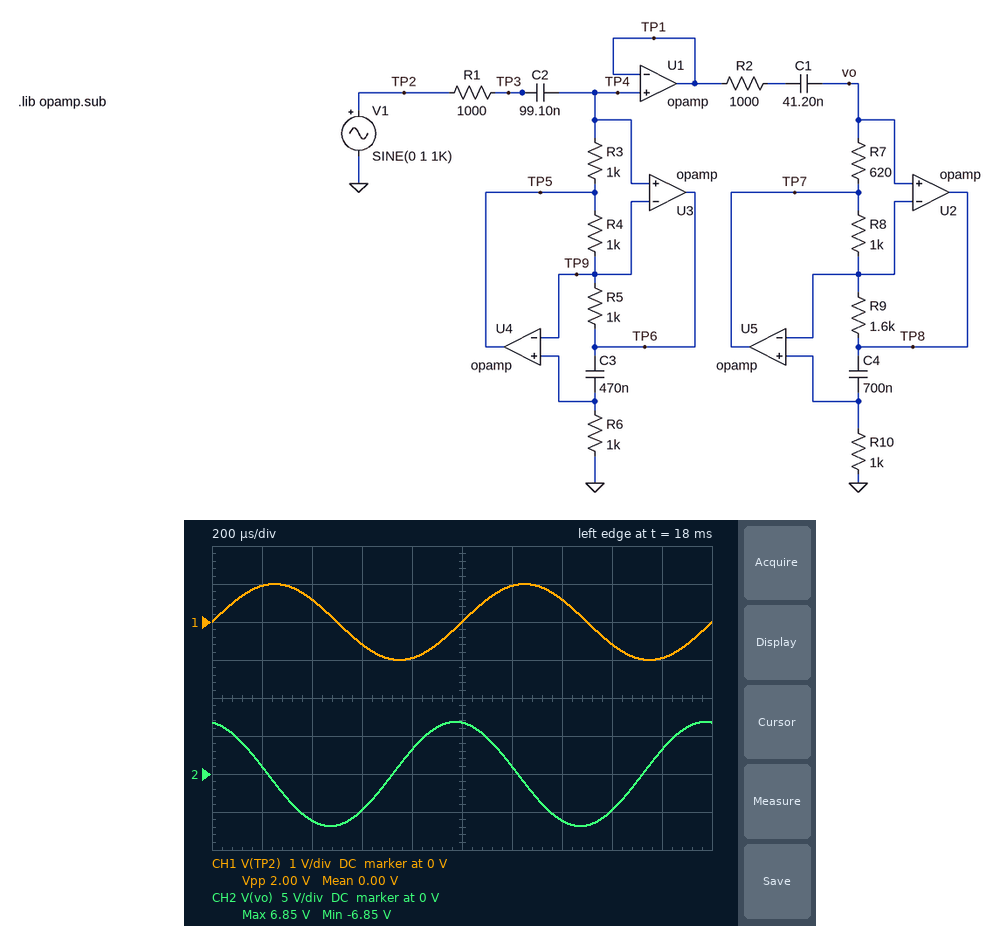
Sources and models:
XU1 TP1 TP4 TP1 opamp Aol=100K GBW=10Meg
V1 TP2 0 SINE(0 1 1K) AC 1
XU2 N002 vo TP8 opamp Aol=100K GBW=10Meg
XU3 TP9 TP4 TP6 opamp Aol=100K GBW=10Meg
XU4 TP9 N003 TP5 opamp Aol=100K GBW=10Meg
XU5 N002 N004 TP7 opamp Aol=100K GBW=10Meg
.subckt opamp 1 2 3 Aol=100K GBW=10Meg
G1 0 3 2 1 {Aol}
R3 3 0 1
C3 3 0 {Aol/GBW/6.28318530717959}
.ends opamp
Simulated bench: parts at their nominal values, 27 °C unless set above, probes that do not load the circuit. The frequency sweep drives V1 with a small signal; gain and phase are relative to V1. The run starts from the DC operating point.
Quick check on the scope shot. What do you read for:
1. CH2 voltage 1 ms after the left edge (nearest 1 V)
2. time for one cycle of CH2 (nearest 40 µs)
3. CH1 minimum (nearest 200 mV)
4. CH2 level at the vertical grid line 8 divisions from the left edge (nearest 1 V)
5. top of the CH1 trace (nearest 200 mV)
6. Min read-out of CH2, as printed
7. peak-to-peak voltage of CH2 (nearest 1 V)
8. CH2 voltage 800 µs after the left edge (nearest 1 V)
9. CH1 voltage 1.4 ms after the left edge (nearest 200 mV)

7 V
1.00 ms
-1.0 V
-5 V
1.0 V
-6.85 V
14 V
3 V
600 mV
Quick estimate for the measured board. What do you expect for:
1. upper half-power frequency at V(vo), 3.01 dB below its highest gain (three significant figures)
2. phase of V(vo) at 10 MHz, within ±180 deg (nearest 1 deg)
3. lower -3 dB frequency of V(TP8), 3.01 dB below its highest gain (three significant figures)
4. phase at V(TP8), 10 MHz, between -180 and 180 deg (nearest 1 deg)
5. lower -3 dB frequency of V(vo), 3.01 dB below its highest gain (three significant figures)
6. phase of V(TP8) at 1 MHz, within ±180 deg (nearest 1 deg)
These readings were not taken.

1.06 kHz
-72 deg
829 Hz
-124 deg
830 Hz
-31 deg
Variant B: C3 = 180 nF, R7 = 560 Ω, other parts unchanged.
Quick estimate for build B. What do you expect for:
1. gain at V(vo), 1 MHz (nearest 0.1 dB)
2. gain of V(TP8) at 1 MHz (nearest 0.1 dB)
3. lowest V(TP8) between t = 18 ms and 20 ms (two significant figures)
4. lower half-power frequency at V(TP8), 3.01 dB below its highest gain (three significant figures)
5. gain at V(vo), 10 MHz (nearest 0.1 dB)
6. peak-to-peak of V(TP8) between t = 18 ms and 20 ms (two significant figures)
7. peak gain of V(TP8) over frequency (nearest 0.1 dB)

-0.9 dB
-0.8 dB
-4.1 V
935 Hz
-20.4 dB
8.2 V
12.7 dB
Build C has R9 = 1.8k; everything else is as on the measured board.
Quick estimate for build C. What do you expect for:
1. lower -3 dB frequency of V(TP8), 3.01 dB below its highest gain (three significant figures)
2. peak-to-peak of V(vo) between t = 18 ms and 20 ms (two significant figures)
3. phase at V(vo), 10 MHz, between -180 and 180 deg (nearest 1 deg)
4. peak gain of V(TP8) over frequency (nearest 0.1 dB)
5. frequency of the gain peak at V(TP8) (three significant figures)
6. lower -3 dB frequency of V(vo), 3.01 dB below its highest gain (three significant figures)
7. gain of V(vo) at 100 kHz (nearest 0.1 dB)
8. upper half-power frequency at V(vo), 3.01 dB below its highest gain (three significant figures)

793 Hz
12 V
-73 deg
19.2 dB
884 Hz
794 Hz
0 dB
989 Hz
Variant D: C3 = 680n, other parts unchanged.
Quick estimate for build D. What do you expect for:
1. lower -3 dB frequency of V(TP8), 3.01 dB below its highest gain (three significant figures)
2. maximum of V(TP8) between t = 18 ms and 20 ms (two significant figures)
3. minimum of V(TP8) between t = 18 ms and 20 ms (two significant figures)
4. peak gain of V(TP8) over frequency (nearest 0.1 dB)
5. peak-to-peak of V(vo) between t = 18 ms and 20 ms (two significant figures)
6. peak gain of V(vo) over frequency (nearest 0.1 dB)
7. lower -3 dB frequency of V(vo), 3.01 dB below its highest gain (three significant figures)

824 Hz
6.0 V
-6.0 V
16.6 dB
12 V
16.3 dB
826 Hz
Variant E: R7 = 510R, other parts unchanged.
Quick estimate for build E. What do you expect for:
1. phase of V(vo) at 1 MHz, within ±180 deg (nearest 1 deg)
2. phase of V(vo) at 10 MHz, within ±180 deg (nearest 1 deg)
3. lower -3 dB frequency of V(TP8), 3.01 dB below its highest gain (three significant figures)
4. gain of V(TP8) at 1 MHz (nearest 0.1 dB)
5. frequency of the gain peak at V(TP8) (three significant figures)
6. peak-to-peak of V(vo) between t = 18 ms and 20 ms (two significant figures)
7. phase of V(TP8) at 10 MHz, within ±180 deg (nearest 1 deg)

-34 deg
-73 deg
898 Hz
-0.8 dB
1.03 kHz
12 V
-125 deg
